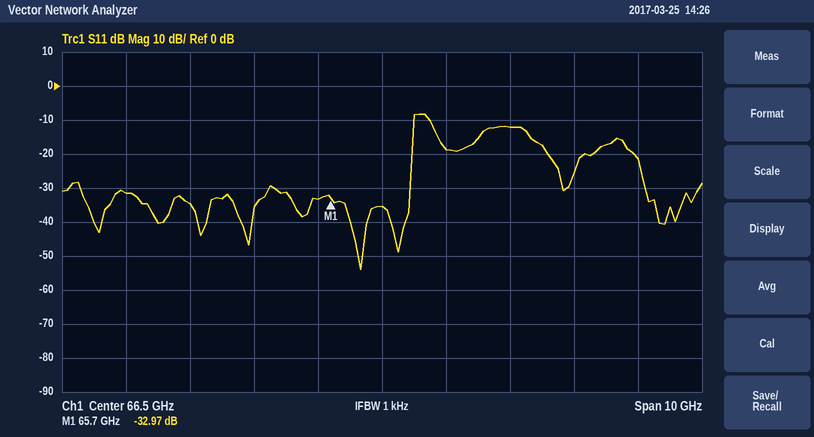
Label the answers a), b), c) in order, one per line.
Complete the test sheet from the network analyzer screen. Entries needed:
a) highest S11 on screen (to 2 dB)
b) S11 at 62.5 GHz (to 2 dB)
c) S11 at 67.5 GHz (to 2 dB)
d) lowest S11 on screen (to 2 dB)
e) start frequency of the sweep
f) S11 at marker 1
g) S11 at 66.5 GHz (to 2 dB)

a) -8 dB
b) -32 dB
c) -18 dB
d) -54 dB
e) 61.5 GHz
f) -32.97 dB
g) -36 dB
